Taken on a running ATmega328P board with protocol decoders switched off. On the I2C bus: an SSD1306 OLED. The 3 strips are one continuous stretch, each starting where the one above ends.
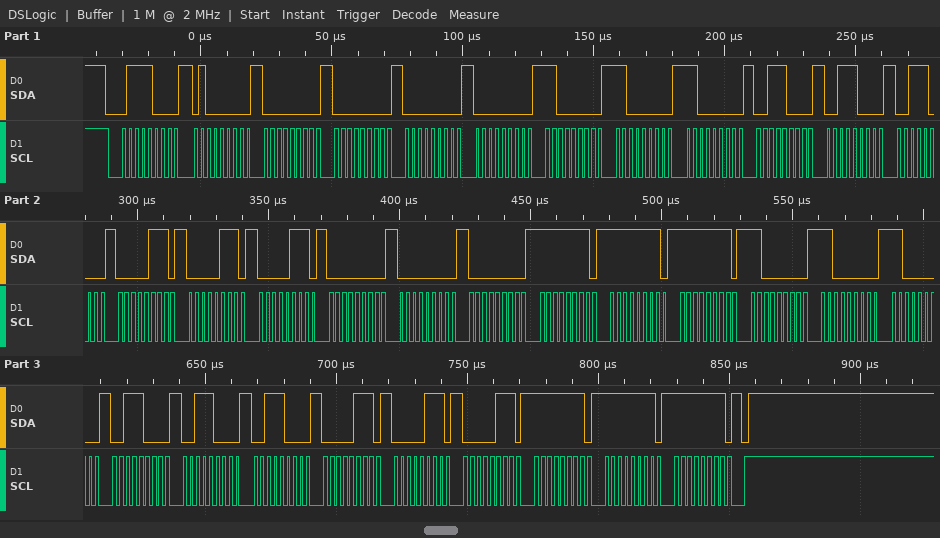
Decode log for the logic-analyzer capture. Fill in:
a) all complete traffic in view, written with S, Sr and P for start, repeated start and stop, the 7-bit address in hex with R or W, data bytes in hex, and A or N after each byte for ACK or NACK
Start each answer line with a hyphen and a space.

- S 3CW A 40 A 00 A 00 A 00 A 00 A C0 A C0 A C0 A 38 A 38 A 38 A 07 A 07 A 07 A 00 A 00 A 00 A FF A FF A FF A C0 A C0 A C0 A 38 A 38 A 38 A 07 A 07 A 07 A FF A FF A FF A P
